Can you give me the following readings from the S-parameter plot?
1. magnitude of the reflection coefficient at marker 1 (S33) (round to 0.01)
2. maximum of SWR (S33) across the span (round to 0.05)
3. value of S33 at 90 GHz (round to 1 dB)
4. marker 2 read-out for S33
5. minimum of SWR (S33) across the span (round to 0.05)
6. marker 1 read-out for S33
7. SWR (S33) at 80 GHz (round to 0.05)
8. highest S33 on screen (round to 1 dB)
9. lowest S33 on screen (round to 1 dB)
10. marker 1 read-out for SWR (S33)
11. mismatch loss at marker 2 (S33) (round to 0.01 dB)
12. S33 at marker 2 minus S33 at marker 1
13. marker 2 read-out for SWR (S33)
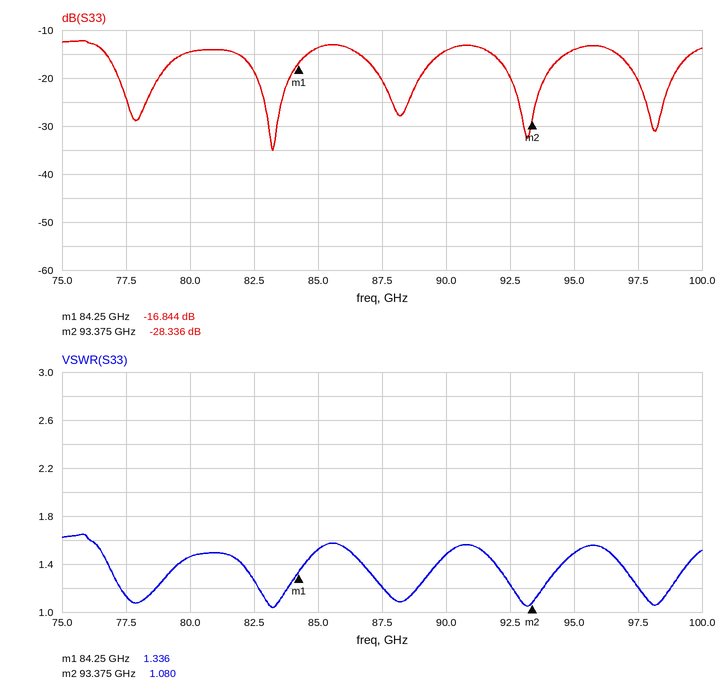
0.14
1.65
-14 dB
-28.336 dB
1.05
-16.844 dB
1.45
-12 dB
-35 dB
1.336
0.01 dB
-11.492 dB
1.080
